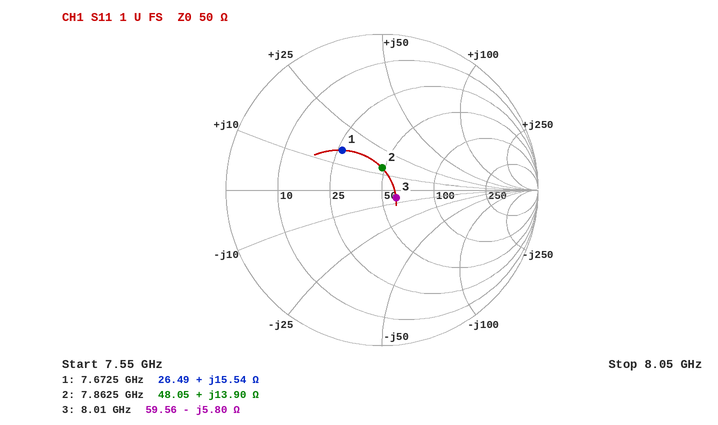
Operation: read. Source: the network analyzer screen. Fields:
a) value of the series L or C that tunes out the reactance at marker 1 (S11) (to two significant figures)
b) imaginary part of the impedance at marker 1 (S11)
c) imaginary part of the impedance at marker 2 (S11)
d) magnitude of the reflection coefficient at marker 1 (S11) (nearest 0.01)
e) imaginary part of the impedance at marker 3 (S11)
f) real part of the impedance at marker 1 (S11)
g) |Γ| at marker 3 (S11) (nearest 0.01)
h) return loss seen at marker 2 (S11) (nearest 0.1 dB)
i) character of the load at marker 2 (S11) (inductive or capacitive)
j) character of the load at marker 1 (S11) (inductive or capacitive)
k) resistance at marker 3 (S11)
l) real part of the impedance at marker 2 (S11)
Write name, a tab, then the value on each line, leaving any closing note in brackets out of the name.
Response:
value of the series L or C that tunes out the reactance at marker 1 (S11)	1.3 pF
imaginary part of the impedance at marker 1	+15.54 Ω
imaginary part of the impedance at marker 2	+13.90 Ω
magnitude of the reflection coefficient at marker 1 (S11)	0.36
imaginary part of the impedance at marker 3	-5.80 Ω
real part of the impedance at marker 1	26.49 Ω
|Γ| at marker 3 (S11)	0.10
return loss seen at marker 2 (S11)	17.0 dB
character of the load at marker 2 (S11)	inductive
character of the load at marker 1 (S11)	inductive
resistance at marker 3	59.56 Ω
real part of the impedance at marker 2	48.05 Ω
